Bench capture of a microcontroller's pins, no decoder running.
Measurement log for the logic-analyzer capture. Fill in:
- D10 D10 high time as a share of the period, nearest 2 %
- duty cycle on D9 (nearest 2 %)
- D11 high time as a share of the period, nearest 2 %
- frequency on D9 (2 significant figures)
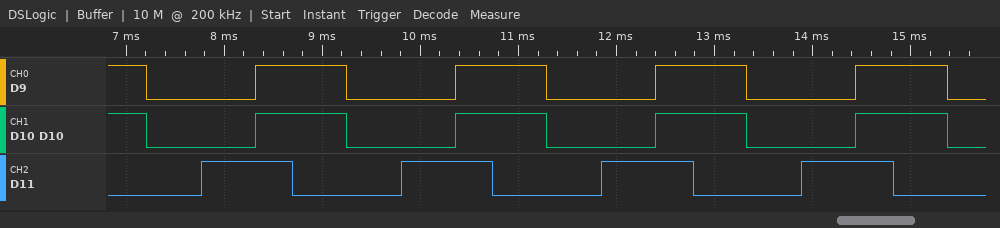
46 %
46 %
46 %
490 Hz
